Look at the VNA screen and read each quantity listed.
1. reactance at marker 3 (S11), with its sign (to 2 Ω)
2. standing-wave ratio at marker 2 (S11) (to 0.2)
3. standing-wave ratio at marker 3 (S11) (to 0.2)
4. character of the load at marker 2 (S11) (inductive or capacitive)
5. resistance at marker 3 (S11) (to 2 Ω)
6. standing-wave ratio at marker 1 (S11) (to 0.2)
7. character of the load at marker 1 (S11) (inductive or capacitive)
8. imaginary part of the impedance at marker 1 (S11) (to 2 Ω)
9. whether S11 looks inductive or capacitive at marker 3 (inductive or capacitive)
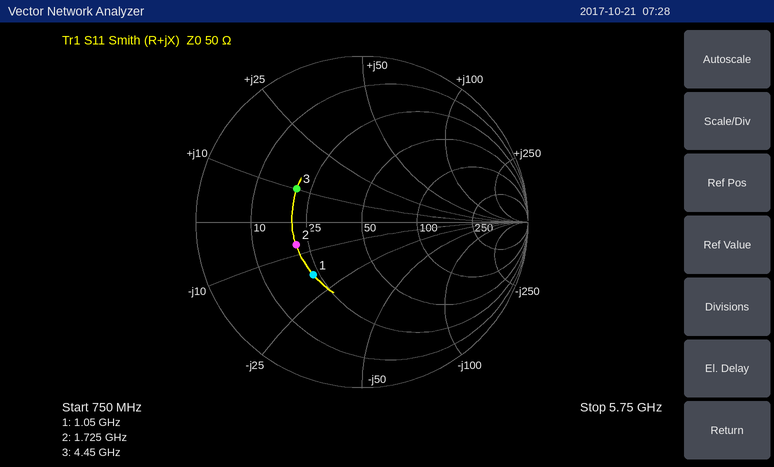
+10 Ω
2.4
2.6
capacitive
20 Ω
2.6
capacitive
-18 Ω
inductive
